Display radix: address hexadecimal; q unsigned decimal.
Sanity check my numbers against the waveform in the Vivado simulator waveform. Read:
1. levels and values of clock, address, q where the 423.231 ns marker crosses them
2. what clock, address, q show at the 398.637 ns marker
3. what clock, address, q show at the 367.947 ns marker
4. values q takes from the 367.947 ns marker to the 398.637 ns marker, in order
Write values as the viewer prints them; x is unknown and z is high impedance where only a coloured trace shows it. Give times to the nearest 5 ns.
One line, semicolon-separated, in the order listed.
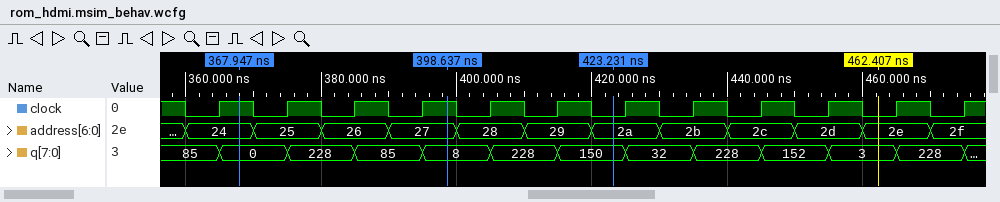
clock=0, address=2a, q=150; clock=1, address=27, q=8; clock=1, address=24, q=0; 0, 228, 85, 8
